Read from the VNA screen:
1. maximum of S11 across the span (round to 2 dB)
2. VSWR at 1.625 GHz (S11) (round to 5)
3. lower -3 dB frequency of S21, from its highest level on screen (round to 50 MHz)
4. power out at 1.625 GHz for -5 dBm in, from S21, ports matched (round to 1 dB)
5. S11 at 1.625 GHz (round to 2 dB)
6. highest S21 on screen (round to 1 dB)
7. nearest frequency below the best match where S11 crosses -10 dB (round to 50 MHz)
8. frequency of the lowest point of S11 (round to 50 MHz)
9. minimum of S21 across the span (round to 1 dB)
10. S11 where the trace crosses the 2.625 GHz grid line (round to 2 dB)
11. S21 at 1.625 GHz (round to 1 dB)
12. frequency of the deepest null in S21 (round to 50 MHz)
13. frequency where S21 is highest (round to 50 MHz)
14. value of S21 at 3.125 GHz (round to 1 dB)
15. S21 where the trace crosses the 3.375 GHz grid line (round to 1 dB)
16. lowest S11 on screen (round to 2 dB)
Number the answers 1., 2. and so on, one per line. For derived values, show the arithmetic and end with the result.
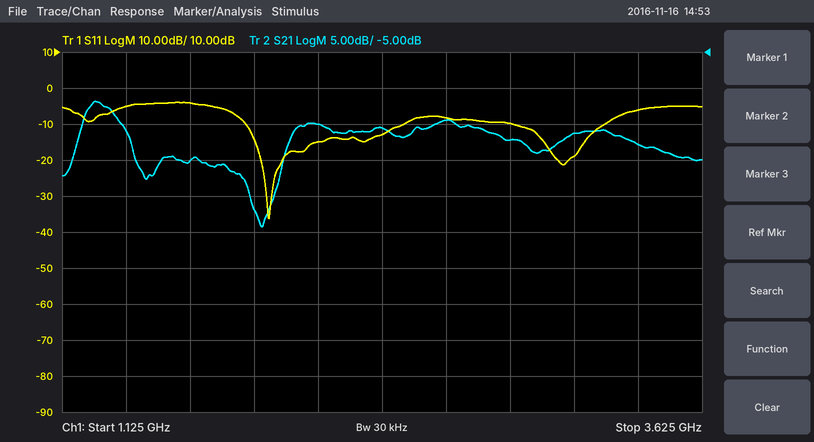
1. -4 dB
2. |Γ| = 10^(-4/20) = 0.6310; VSWR = (1 + 0.6310)/(1 − 0.6310) ≈ 4.42, so 5 to the nearest 5
3. 1.20 GHz
4. -5 dBm + (-20 dB) = -25 dBm
5. -4 dB
6. -12 dB
7. 1.85 GHz
8. 1.95 GHz
9. -29 dB
10. -8 dB
11. -20 dB
12. 1.90 GHz
13. 1.25 GHz
14. -16 dB
15. -18 dB
16. -36 dB
